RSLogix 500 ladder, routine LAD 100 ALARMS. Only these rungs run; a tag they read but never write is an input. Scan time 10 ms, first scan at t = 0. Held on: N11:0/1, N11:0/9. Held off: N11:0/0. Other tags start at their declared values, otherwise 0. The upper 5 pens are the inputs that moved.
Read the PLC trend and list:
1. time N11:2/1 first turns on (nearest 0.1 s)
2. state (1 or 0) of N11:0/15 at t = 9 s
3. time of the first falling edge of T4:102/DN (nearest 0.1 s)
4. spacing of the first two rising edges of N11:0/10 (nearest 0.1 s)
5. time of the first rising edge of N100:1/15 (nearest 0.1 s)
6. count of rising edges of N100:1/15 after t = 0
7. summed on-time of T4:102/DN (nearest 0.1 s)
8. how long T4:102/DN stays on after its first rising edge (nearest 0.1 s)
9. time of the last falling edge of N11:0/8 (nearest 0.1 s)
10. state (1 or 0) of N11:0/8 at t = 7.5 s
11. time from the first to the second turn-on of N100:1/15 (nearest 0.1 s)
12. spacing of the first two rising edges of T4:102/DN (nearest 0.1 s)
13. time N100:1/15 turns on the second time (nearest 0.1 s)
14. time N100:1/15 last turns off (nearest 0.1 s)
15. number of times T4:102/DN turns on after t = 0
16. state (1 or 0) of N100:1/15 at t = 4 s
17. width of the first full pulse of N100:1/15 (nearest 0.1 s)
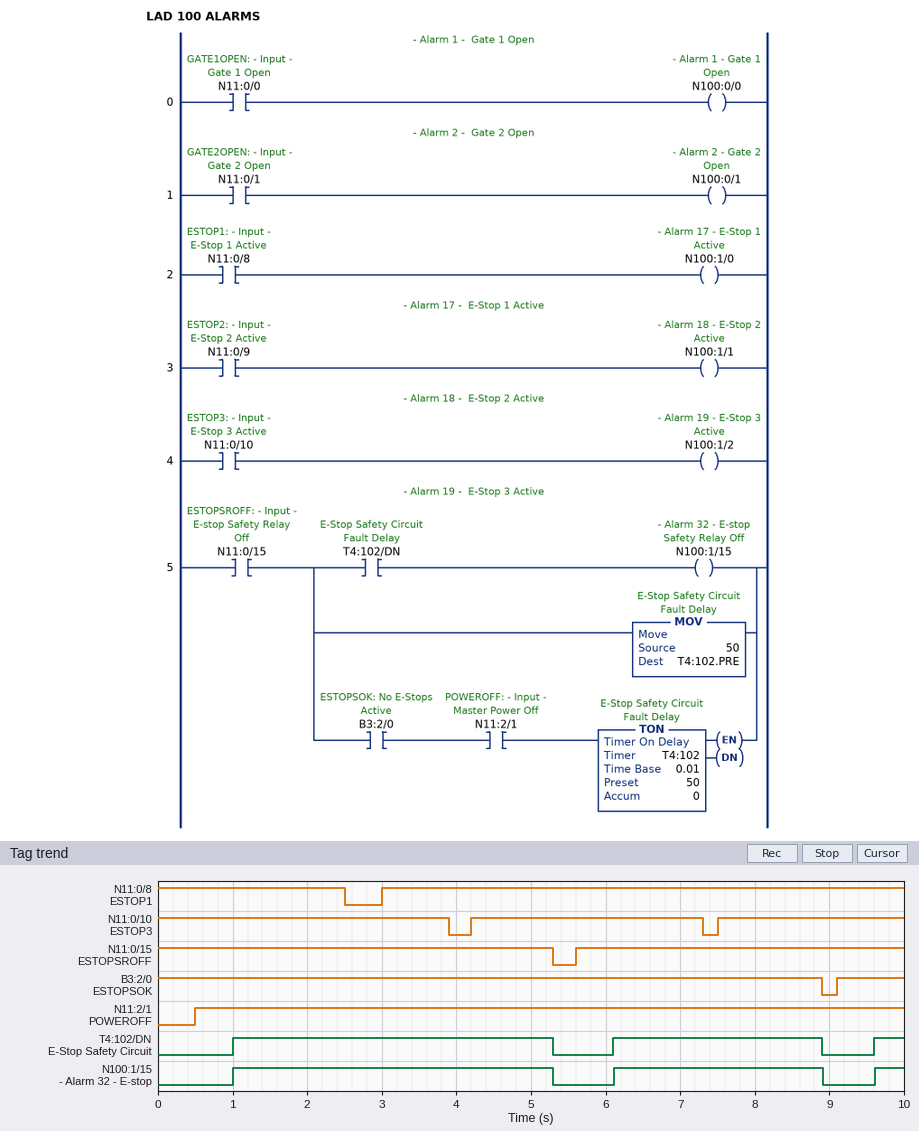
0.5 s
1
5.3 s
3.3 s
1.0 s
3
7.5 s
4.3 s
2.5 s
1
5.1 s
5.1 s
6.1 s
8.9 s
3
1
4.3 s
